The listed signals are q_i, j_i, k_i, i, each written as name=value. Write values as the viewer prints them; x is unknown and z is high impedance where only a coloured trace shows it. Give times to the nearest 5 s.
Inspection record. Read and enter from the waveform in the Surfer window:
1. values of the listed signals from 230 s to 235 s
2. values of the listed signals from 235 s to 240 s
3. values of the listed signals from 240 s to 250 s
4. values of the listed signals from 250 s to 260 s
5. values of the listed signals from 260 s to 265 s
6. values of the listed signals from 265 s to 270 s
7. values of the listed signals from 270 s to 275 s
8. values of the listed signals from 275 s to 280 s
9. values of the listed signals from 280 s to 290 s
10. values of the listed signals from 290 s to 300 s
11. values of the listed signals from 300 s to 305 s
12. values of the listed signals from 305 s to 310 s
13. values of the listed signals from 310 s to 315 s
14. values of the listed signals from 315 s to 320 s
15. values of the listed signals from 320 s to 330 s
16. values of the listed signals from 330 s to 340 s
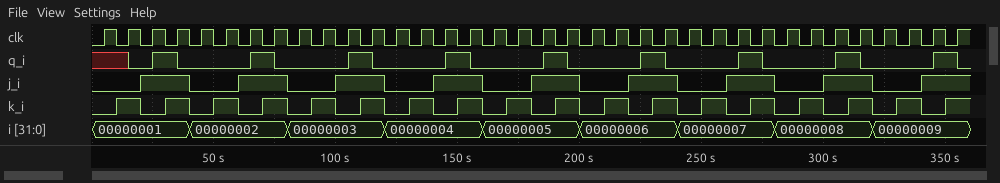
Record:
q_i=1, j_i=1, k_i=1, i=00000006
q_i=0, j_i=1, k_i=1, i=00000006
q_i=0, j_i=0, k_i=0, i=00000007
q_i=0, j_i=0, k_i=1, i=00000007
q_i=0, j_i=1, k_i=0, i=00000007
q_i=1, j_i=1, k_i=0, i=00000007
q_i=1, j_i=1, k_i=1, i=00000007
q_i=0, j_i=1, k_i=1, i=00000007
q_i=0, j_i=0, k_i=0, i=00000008
q_i=0, j_i=0, k_i=1, i=00000008
q_i=0, j_i=1, k_i=0, i=00000008
q_i=1, j_i=1, k_i=0, i=00000008
q_i=1, j_i=1, k_i=1, i=00000008
q_i=0, j_i=1, k_i=1, i=00000008
q_i=0, j_i=0, k_i=0, i=00000009
q_i=0, j_i=0, k_i=1, i=00000009
